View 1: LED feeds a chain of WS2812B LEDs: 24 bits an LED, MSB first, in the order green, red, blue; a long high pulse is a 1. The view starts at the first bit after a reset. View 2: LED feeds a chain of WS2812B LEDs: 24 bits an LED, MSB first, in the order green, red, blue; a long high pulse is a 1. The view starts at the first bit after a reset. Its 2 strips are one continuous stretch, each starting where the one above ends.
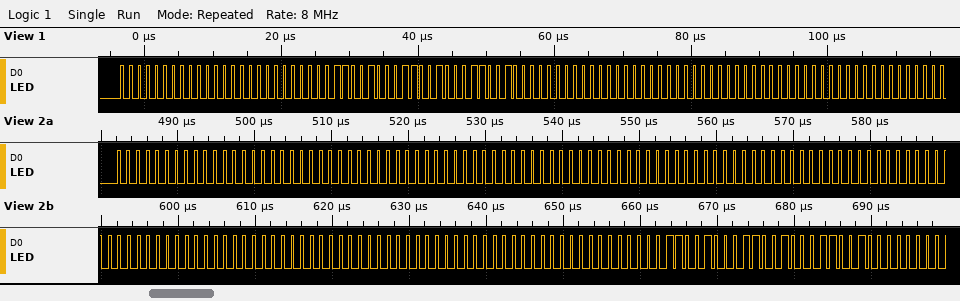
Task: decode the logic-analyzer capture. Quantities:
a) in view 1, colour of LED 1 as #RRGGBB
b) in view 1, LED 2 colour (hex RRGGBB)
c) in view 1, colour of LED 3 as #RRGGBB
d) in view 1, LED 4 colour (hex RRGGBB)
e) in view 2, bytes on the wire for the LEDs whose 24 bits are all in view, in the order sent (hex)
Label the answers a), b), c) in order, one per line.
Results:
a) #000000
b) #646464
c) #000000
d) #000000
e) 00 00 00 00 00 00 00 00 00 00 00 00 00 00 00 00 00 00 64 64 64
